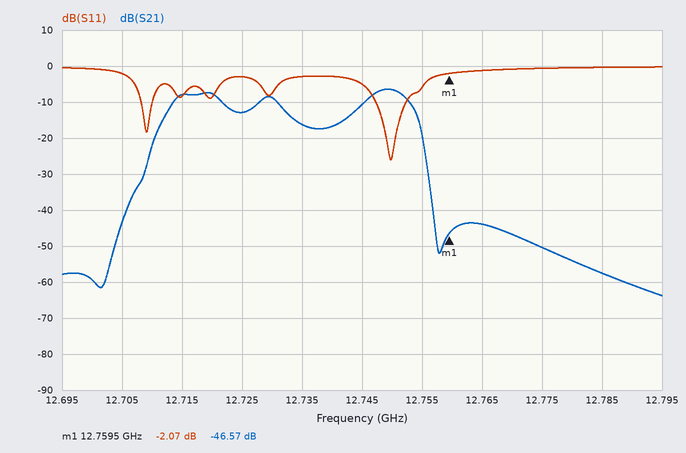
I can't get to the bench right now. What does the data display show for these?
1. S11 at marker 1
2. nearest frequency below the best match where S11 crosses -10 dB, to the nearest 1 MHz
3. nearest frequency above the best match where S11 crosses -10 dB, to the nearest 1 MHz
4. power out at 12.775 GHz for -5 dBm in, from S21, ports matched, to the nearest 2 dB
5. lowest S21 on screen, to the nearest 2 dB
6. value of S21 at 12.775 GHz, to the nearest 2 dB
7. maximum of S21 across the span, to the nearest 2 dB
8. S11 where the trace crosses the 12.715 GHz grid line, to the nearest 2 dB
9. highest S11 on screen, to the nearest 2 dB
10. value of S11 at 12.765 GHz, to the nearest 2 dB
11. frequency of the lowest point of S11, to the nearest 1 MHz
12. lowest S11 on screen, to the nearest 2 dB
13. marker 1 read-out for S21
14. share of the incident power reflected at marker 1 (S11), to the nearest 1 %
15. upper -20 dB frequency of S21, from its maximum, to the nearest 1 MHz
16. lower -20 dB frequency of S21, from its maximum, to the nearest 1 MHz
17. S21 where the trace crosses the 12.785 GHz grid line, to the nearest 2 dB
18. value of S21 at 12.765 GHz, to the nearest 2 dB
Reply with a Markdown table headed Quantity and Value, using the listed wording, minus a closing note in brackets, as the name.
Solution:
| Quantity | Value |
|---|---|
| S11 at marker 1 | -2.07 dB |
| nearest frequency below the best match where S11 crosses -10 dB, to the nearest 1 MHz | 12.747 GHz |
| nearest frequency above the best match where S11 crosses -10 dB, to the nearest 1 MHz | 12.752 GHz |
| power out at 12.775 GHz for -5 dBm in, from S21, ports matched, to the nearest 2 dB | -56 dBm |
| lowest S21 on screen, to the nearest 2 dB | -64 dB |
| value of S21 at 12.775 GHz, to the nearest 2 dB | -50 dB |
| maximum of S21 across the span, to the nearest 2 dB | -6 dB |
| S11 where the trace crosses the 12.715 GHz grid line, to the nearest 2 dB | -8 dB |
| highest S11 on screen, to the nearest 2 dB | 0 dB |
| value of S11 at 12.765 GHz, to the nearest 2 dB | -2 dB |
| frequency of the lowest point of S11, to the nearest 1 MHz | 12.750 GHz |
| lowest S11 on screen, to the nearest 2 dB | -26 dB |
| marker 1 read-out for S21 | -46.57 dB |
| share of the incident power reflected at marker 1 (S11), to the nearest 1 % | 62 % |
| upper -20 dB frequency of S21, from its maximum, to the nearest 1 MHz | 12.756 GHz |
| lower -20 dB frequency of S21, from its maximum, to the nearest 1 MHz | 12.709 GHz |
| S21 where the trace crosses the 12.785 GHz grid line, to the nearest 2 dB | -58 dB |
| value of S21 at 12.765 GHz, to the nearest 2 dB | -44 dB |
